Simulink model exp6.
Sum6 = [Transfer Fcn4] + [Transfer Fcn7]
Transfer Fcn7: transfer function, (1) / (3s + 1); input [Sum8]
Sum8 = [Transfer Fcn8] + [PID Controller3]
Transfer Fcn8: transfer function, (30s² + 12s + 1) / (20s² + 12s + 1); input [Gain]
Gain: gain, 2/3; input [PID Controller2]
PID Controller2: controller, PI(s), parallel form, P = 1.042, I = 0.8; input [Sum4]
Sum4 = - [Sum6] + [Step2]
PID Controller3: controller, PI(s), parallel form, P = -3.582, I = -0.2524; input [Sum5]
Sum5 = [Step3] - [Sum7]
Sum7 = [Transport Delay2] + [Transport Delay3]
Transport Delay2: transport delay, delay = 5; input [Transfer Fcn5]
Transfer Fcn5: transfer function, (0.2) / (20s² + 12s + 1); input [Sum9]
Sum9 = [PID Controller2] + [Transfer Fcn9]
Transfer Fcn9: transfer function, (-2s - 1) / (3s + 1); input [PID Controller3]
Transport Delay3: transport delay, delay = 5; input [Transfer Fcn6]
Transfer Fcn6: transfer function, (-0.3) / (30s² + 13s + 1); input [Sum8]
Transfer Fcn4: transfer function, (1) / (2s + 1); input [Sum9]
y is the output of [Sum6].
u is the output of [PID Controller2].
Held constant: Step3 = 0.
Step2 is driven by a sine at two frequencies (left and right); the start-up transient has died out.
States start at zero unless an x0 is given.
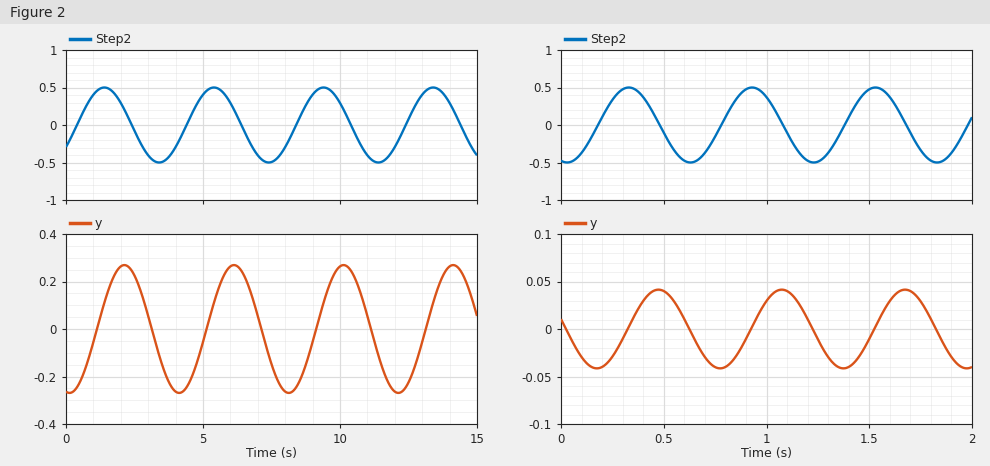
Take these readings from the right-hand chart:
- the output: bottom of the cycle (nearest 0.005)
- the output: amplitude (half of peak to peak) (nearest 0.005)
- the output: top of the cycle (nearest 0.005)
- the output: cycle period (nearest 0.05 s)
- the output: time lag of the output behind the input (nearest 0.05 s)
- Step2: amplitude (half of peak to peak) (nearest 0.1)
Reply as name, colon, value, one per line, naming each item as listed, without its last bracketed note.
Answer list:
the output: bottom of the cycle: -0.040
the output: amplitude (half of peak to peak): 0.040
the output: top of the cycle: 0.040
the output: cycle period: 0.60 s
the output: time lag of the output behind the input: 0.15 s
Step2: amplitude (half of peak to peak): 0.5
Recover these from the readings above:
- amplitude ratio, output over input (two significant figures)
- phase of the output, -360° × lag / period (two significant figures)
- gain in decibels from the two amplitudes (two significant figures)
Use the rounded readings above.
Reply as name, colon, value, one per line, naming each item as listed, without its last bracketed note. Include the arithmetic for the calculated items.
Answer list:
amplitude ratio, output over input: 0.04 / 0.5 = 0.080
phase of the output, -360° × lag / period: -360 × 0.15 / 0.6 = -90°
gain in decibels from the two amplitudes: 20 log10(0.04 / 0.5) = -22 dB
